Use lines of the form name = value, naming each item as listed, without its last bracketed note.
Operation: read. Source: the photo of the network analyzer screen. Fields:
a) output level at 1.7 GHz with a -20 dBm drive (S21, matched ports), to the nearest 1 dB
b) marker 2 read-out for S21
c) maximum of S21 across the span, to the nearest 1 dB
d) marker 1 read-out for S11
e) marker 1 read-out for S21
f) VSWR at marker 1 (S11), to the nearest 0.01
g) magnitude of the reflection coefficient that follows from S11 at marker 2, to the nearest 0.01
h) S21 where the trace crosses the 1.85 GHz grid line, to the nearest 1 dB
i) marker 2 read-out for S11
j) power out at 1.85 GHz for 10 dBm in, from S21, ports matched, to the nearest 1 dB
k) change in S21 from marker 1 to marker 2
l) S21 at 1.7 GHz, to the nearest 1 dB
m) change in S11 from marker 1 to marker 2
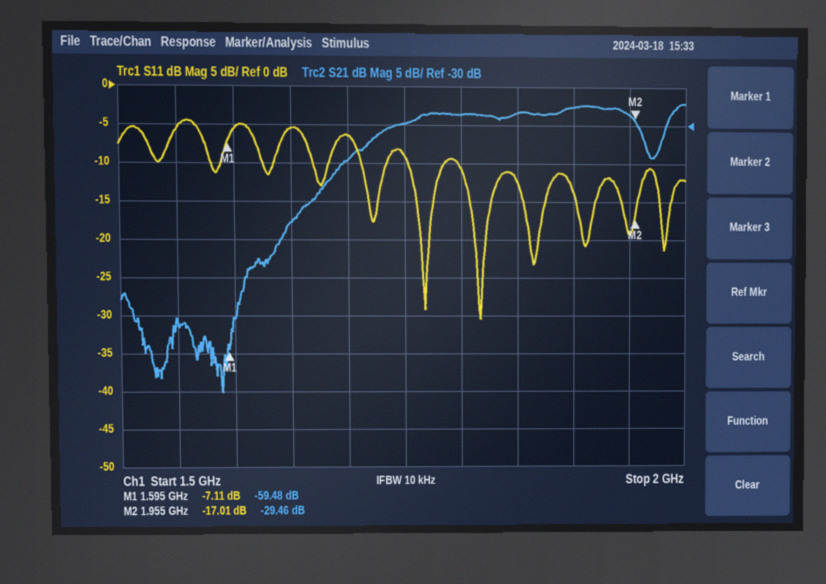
output level at 1.7 GHz with a -20 dBm drive (S21, matched ports), to the nearest 1 dB = -55 dBm
marker 2 read-out for S21 = -29.46 dB
maximum of S21 across the span, to the nearest 1 dB = -27 dB
marker 1 read-out for S11 = -7.11 dB
marker 1 read-out for S21 = -59.48 dB
VSWR at marker 1 (S11), to the nearest 0.01 = 2.58
magnitude of the reflection coefficient that follows from S11 at marker 2, to the nearest 0.01 = 0.14
S21 where the trace crosses the 1.85 GHz grid line, to the nearest 1 dB = -28 dB
marker 2 read-out for S11 = -17.01 dB
power out at 1.85 GHz for 10 dBm in, from S21, ports matched, to the nearest 1 dB = -18 dBm
change in S21 from marker 1 to marker 2 = 30.02 dB
S21 at 1.7 GHz, to the nearest 1 dB = -35 dB
change in S11 from marker 1 to marker 2 = -9.90 dB
